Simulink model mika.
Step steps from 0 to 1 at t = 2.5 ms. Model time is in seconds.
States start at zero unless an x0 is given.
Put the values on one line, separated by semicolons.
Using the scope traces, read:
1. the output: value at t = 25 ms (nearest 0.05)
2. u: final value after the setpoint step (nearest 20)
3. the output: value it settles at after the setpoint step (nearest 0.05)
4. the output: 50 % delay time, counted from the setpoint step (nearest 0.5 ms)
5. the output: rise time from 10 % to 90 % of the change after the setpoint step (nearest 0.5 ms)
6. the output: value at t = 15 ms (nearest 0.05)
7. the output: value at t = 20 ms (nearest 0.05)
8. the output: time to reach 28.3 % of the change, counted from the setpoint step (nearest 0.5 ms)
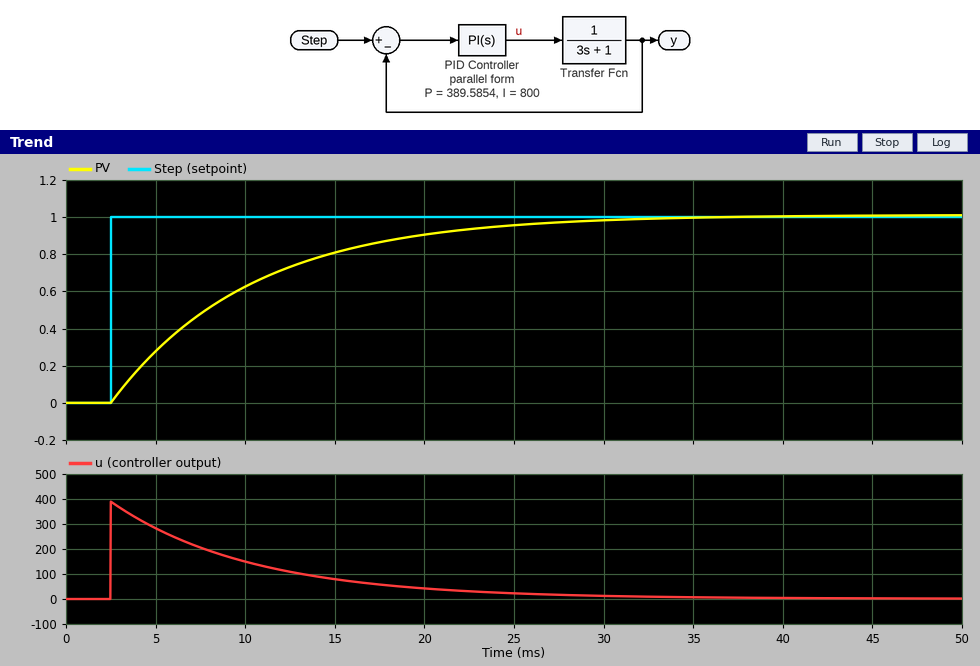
0.95; 0; 1.00; 5.5 ms; 17.0 ms; 0.80; 0.90; 2.5 ms
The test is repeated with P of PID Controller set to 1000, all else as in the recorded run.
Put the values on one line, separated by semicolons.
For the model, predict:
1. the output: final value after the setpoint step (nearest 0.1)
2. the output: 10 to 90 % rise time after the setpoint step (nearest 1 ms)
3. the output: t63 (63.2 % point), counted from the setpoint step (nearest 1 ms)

1.0; 7 ms; 3 ms
